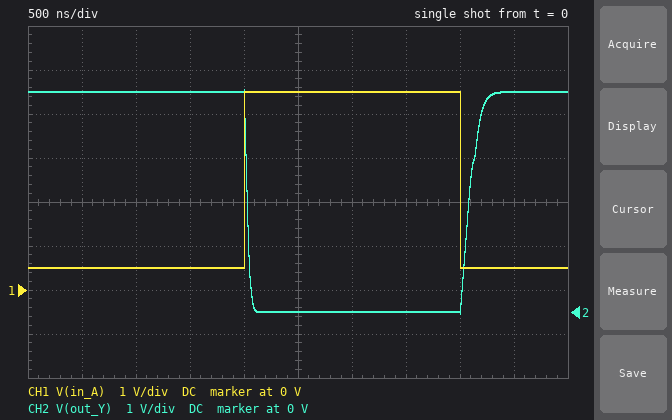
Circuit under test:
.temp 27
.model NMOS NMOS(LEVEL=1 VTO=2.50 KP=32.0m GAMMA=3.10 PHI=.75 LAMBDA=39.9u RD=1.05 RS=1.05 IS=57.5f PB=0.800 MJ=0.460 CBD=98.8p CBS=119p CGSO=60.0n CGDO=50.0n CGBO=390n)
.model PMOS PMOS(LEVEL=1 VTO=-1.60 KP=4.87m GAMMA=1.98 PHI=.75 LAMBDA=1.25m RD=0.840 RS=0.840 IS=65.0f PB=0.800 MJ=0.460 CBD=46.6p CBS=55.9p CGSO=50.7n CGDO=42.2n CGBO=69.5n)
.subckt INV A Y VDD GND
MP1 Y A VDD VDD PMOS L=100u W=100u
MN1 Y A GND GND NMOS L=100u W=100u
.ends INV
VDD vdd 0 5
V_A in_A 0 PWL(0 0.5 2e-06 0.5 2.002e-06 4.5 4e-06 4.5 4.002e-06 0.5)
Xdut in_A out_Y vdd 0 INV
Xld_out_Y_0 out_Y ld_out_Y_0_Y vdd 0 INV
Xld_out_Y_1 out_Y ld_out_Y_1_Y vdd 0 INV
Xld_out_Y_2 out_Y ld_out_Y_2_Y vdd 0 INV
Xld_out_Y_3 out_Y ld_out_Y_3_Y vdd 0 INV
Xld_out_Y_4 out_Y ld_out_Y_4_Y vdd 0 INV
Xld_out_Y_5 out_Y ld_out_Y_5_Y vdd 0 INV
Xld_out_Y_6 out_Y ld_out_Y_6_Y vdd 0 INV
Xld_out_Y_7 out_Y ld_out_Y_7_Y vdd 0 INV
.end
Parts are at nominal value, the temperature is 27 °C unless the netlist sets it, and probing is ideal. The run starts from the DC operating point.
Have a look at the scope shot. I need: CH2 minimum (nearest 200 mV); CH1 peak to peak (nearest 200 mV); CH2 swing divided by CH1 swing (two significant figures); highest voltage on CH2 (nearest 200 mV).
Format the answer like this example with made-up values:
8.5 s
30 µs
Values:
0 V
4.0 V
1.3
5.0 V
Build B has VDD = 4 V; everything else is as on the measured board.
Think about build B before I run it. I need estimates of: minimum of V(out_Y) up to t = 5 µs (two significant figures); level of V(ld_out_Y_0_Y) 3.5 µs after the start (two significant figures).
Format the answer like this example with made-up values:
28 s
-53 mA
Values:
-50 mV
4.0 V
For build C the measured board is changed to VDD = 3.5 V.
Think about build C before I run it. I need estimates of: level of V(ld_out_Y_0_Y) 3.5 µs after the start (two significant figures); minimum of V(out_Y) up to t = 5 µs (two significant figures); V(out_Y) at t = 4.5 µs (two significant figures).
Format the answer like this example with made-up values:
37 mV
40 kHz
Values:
3.5 V
-53 mV
3.0 V
